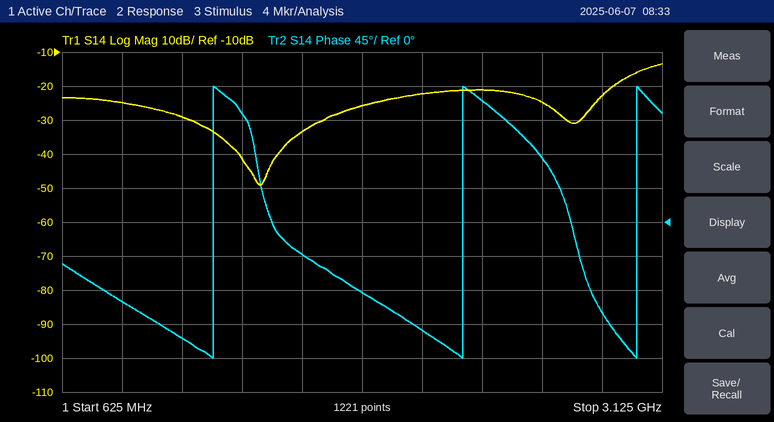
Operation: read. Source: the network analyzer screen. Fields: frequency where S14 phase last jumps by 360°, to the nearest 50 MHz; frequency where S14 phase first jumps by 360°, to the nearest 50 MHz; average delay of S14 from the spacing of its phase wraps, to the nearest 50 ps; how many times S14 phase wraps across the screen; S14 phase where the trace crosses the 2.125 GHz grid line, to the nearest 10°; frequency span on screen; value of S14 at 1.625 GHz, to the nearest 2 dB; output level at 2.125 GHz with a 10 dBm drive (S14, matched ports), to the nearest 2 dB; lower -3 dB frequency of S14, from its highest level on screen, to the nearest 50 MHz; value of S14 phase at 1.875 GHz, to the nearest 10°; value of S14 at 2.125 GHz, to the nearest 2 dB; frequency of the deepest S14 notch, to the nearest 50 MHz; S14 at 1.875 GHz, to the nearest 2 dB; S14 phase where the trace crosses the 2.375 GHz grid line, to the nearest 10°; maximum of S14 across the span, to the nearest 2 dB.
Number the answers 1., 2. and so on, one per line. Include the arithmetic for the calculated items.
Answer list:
1. 3.00 GHz
2. 1.25 GHz
3. 2 cycles / (3.00 GHz − 1.25 GHz) ≈ 1.14 ns, so 1.15 ns to the nearest 50 ps
4. 3
5. -140°
6. 2.5 GHz
7. -34 dB
8. 10 dBm + (-22 dB) = -12 dBm
9. 3.00 GHz
10. -90°
11. -22 dB
12. 1.45 GHz
13. -26 dB
14. 160°
15. -14 dB
